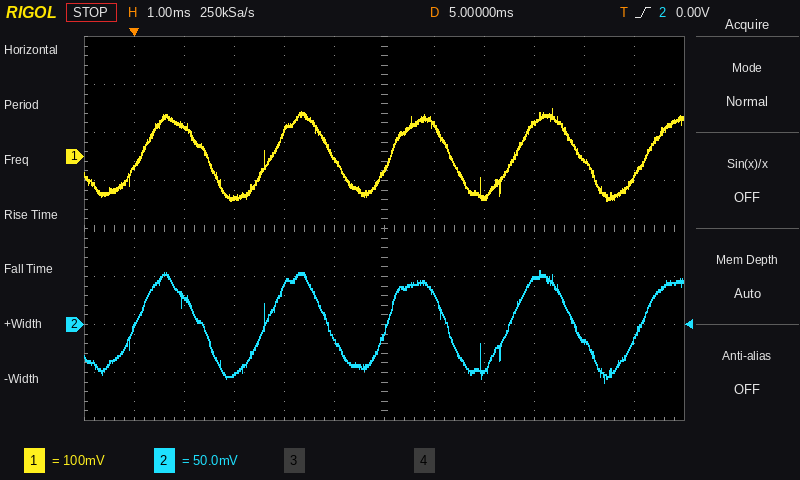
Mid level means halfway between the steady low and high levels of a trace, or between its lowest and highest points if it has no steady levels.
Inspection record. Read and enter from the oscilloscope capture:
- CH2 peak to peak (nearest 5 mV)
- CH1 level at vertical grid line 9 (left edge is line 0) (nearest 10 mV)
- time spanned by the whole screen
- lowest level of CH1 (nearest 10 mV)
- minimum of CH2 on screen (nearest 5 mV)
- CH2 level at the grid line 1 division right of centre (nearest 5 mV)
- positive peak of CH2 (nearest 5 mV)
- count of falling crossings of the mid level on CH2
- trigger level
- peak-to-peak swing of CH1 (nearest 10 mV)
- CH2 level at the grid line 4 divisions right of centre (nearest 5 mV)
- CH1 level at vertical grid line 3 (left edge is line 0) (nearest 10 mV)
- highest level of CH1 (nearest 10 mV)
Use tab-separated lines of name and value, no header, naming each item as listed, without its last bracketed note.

CH2 peak to peak	115 mV
CH1 level at vertical grid line 9 (left edge is line 0)	70 mV
time spanned by the whole screen	12 ms
lowest level of CH1	-90 mV
minimum of CH2 on screen	-60 mV
CH2 level at the grid line 1 division right of centre	30 mV
positive peak of CH2	55 mV
count of falling crossings of the mid level on CH2	4
trigger level	0.00 V
peak-to-peak swing of CH1	190 mV
CH2 level at the grid line 4 divisions right of centre	-15 mV
CH1 level at vertical grid line 3 (left edge is line 0)	-90 mV
highest level of CH1	100 mV
